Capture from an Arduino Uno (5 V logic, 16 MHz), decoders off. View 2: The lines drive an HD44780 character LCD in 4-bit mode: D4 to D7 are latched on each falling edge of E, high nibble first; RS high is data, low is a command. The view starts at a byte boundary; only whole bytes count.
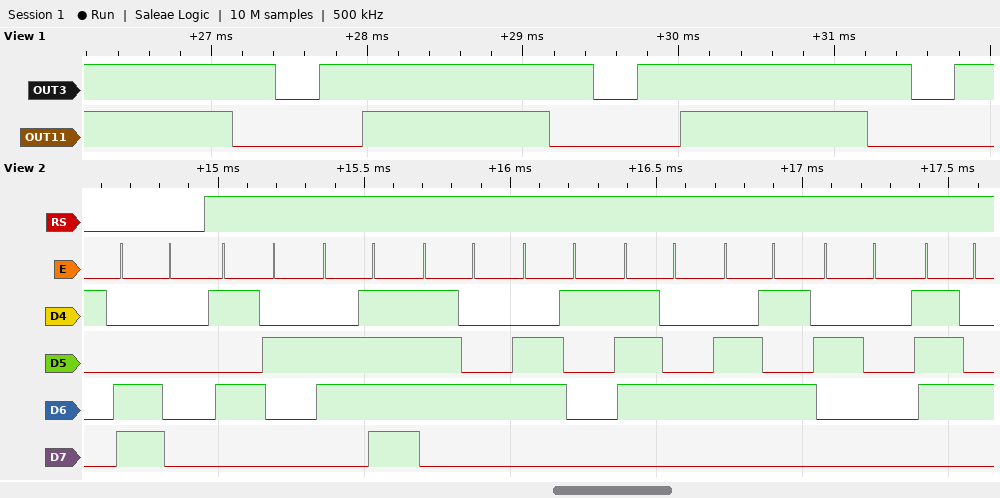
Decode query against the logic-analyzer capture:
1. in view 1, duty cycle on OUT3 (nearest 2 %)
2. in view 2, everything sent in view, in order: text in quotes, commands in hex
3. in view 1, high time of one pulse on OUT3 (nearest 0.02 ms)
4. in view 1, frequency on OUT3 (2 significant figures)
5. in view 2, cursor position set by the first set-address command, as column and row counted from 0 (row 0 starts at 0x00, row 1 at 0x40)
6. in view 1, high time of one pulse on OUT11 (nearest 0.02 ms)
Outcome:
86 %
0xC0 "Rotate t"
1.76 ms
490 Hz
column 0, row 1
1.20 ms
